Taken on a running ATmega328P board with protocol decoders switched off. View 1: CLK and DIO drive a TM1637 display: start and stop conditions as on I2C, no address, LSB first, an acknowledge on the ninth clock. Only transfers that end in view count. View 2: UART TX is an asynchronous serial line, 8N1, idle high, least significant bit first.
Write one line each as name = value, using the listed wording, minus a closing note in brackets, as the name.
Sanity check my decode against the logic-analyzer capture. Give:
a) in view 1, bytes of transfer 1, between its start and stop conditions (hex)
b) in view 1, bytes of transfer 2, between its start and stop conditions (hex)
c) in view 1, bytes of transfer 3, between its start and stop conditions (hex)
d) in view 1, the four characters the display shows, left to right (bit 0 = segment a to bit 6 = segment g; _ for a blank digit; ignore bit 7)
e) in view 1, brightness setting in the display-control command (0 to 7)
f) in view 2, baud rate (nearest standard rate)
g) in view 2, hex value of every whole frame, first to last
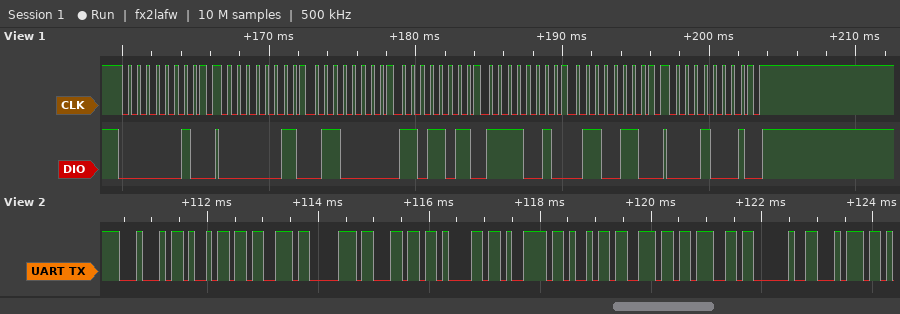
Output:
in view 1, bytes of transfer 1, between its start and stop conditions = 40
in view 1, bytes of transfer 2, between its start and stop conditions = C0 06 DB 4F 66
in view 1, bytes of transfer 3, between its start and stop conditions = 88
in view 1, the four characters the display shows, left to right = 1234
in view 1, brightness setting in the display-control command = 0
in view 2, baud rate = 9600 baud
in view 2, hex value of every whole frame, first to last = 44 69 73 70 6C 61 79 69 6E 67 20 74
